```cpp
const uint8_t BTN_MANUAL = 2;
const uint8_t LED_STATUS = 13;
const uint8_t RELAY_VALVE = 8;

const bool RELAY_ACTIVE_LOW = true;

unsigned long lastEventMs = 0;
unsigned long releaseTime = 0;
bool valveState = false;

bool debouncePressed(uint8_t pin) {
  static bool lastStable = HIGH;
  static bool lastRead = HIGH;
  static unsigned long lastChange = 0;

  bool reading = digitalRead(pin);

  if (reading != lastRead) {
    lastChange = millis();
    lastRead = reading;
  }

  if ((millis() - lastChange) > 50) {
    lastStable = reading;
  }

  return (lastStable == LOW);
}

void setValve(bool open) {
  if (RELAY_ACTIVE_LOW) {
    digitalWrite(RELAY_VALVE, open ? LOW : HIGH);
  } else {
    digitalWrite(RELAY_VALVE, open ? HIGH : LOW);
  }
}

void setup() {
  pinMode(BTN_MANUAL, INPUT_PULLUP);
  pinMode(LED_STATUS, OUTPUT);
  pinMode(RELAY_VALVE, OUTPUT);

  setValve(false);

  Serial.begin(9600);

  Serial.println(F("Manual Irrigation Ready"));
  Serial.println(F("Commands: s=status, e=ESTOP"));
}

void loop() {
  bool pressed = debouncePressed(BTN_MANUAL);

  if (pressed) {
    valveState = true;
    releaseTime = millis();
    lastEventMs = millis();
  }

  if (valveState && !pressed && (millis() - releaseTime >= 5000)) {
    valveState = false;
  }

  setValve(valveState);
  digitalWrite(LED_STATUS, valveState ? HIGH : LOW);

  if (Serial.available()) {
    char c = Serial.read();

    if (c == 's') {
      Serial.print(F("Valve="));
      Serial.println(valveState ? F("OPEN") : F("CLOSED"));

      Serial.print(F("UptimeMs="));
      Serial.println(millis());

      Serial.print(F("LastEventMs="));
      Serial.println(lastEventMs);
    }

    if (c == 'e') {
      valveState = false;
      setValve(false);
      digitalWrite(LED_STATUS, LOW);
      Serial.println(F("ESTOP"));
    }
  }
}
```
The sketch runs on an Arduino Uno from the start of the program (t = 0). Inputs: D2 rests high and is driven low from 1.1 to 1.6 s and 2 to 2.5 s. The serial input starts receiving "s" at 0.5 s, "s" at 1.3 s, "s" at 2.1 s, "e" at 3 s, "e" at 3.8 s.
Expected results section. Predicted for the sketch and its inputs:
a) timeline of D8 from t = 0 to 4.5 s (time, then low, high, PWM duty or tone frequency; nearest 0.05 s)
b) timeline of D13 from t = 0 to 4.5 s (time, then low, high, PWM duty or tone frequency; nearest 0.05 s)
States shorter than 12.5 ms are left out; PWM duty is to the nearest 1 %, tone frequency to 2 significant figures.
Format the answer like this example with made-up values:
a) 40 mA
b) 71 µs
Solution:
a) 0 s high; 1.15 s low; 3 s high
b) 0 s low; 1.15 s high; 3 s low
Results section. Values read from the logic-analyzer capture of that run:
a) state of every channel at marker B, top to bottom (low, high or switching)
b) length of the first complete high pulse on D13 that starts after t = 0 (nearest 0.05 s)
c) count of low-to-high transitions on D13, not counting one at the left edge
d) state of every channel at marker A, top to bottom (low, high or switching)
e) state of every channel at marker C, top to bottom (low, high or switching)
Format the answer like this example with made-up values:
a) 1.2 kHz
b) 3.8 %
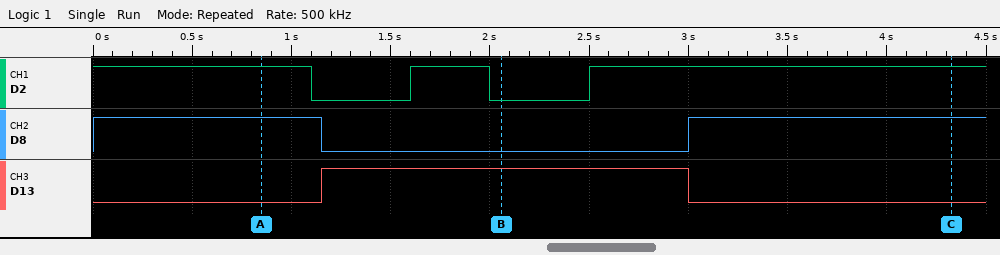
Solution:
a) D2 low, D8 low, D13 high
b) 1.85 s
c) 1
d) D2 high, D8 high, D13 low
e) D2 high, D8 high, D13 low
